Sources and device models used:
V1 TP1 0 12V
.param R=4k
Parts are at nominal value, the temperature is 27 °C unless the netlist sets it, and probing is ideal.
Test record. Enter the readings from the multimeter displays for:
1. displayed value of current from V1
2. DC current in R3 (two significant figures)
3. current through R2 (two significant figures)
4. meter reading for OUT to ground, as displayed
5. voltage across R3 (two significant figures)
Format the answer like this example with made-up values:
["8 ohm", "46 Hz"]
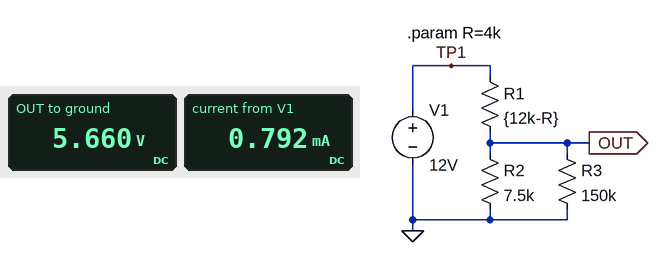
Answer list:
["0.792 mA", "38 µA", "750 µA", "5.660 V", "5.7 V"]
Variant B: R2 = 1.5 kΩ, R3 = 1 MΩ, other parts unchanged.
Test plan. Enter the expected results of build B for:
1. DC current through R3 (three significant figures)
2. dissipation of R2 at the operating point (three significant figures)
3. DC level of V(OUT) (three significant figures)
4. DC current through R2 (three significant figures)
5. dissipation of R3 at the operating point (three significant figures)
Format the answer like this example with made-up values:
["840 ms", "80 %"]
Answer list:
["1.89 µA", "2.39 mW", "1.89 V", "1.26 mA", "3.58 µW"]
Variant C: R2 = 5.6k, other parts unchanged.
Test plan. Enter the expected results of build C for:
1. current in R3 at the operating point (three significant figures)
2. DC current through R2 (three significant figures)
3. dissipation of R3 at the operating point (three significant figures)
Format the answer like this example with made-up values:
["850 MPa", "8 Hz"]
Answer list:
["32.2 µA", "863 µA", "156 µW"]
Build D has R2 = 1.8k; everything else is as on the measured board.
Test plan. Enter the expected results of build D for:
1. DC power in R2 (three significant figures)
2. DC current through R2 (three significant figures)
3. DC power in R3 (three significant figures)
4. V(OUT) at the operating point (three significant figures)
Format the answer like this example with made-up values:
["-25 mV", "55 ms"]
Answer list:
["2.65 mW", "1.21 mA", "31.8 µW", "2.18 V"]
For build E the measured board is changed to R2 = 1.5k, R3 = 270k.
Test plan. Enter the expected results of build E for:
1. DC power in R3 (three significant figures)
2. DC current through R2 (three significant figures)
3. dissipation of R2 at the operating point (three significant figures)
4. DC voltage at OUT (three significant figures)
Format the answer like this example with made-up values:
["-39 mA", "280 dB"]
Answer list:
["13.2 µW", "1.26 mA", "2.37 mW", "1.89 V"]
